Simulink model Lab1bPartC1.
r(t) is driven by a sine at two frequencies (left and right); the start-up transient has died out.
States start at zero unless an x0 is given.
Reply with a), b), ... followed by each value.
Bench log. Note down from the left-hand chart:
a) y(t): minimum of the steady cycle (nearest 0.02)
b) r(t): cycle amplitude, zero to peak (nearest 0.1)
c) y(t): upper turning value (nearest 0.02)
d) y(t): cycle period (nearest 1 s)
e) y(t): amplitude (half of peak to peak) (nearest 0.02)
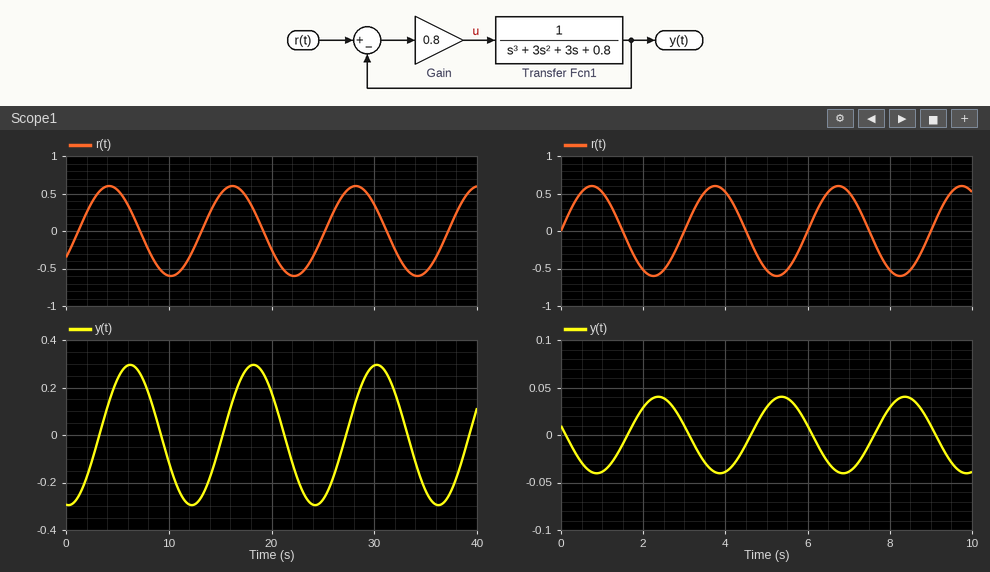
a) -0.30
b) 0.6
c) 0.30
d) 12 s
e) 0.30
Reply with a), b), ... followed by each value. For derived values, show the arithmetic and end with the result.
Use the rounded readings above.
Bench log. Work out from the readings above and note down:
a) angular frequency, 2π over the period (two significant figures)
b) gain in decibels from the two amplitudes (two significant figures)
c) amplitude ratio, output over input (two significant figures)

a) 2π / 12 = 0.52 rad/s
b) 20 log10(0.3 / 0.6) = -6.0 dB
c) 0.3 / 0.6 = 0.50
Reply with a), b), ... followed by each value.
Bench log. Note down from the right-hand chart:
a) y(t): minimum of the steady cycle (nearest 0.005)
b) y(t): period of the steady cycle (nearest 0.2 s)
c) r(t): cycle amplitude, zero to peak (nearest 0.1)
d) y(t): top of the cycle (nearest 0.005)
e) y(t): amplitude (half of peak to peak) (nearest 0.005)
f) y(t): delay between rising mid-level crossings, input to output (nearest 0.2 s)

a) -0.040
b) 3.0 s
c) 0.6
d) 0.040
e) 0.040
f) 1.6 s
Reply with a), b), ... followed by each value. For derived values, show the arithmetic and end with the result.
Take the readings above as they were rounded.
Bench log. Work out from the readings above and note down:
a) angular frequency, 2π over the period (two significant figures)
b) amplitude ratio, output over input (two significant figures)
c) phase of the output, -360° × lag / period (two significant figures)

a) 2π / 3 = 2.1 rad/s
b) 0.04 / 0.6 = 0.067
c) -360 × 1.6 / 3 = -190°
